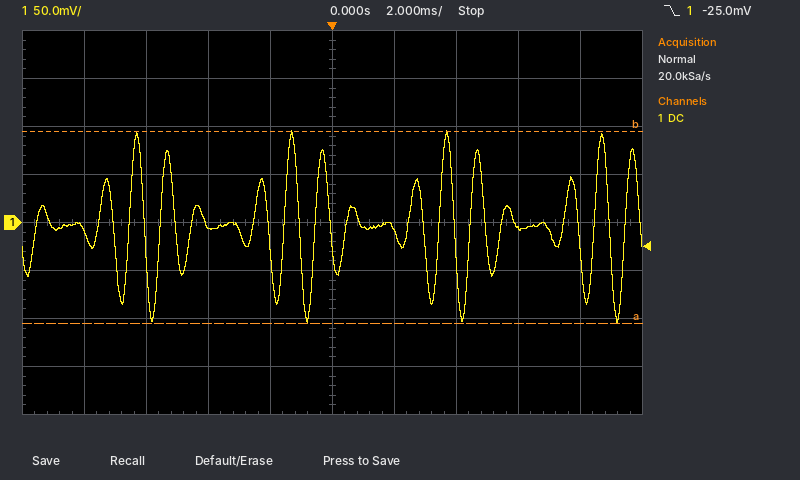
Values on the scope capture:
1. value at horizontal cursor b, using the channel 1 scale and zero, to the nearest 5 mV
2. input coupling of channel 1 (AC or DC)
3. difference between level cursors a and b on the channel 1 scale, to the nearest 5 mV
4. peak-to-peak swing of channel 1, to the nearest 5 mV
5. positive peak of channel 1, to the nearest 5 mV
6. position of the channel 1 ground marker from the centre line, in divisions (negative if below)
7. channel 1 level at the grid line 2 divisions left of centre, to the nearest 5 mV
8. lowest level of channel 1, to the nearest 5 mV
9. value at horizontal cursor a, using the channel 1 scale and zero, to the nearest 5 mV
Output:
95 mV
DC
200 mV
200 mV
95 mV
0.0 div
-5 mV
-105 mV
-105 mV
